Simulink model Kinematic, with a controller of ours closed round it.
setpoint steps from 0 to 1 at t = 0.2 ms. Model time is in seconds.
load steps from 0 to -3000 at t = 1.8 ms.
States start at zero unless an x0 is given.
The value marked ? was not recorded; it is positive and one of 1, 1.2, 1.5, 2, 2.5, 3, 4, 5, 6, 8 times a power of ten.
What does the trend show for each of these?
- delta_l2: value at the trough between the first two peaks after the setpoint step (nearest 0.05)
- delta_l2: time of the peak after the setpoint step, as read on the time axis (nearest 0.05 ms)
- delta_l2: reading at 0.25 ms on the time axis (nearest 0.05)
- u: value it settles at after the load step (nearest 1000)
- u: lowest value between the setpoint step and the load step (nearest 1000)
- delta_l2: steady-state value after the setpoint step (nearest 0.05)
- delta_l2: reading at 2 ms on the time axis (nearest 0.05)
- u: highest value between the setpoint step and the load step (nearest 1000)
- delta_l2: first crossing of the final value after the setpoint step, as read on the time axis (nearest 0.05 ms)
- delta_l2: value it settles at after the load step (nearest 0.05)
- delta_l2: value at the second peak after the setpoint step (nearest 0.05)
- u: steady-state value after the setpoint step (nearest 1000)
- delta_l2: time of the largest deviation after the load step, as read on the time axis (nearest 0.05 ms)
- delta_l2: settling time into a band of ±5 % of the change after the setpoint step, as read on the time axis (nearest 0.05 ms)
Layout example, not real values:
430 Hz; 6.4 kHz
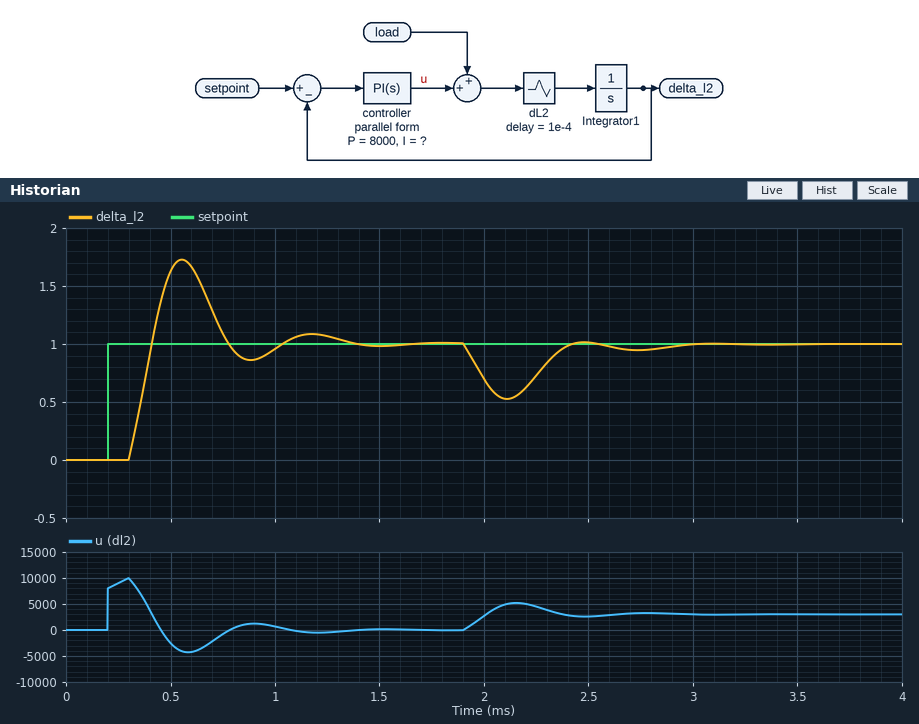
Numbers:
0.85; 0.55 ms; 0.00; 3000; -4000; 1.00; 0.70; 10000; 0.40 ms; 1.00; 1.10; 0; 2.10 ms; 1.30 ms
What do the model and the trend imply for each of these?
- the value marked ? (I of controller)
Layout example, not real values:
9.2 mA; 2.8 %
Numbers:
2e+07
